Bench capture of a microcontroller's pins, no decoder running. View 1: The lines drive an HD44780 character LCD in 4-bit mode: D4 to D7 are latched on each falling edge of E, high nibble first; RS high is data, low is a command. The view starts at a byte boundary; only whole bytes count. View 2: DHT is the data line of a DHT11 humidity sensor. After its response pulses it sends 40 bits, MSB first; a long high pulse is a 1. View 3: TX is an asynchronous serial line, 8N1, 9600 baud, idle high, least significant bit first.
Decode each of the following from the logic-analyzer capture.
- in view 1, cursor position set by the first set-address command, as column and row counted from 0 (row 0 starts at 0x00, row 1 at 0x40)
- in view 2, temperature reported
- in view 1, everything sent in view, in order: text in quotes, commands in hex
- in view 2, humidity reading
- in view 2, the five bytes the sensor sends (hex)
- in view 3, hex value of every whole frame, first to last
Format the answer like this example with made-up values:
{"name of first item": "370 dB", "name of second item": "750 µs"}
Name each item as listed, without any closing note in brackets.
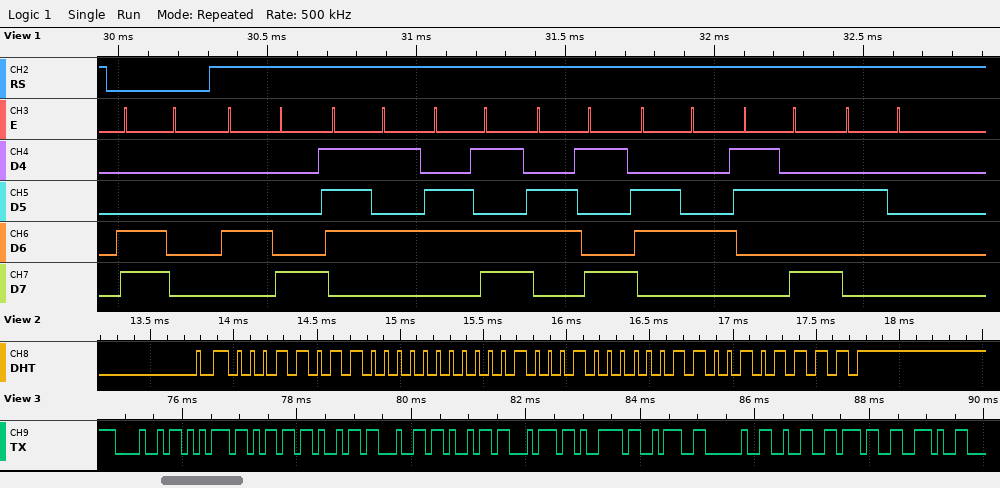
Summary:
{"in view 1, cursor position set by the first set-address command, as column and row counted from 0": "column 0, row 1", "in view 2, temperature reported": "17.3 °C", "in view 1, everything sent in view, in order: text in quotes, commands in hex": "0xC0 \"Humid: \"", "in view 2, humidity reading": "27 %", "in view 2, the five bytes the sensor sends": "1B 00 11 03 2F", "in view 3, hex value of every whole frame, first to last": "48 75 6D 69 64 69 74 79 3A 20 32 37 2E"}
